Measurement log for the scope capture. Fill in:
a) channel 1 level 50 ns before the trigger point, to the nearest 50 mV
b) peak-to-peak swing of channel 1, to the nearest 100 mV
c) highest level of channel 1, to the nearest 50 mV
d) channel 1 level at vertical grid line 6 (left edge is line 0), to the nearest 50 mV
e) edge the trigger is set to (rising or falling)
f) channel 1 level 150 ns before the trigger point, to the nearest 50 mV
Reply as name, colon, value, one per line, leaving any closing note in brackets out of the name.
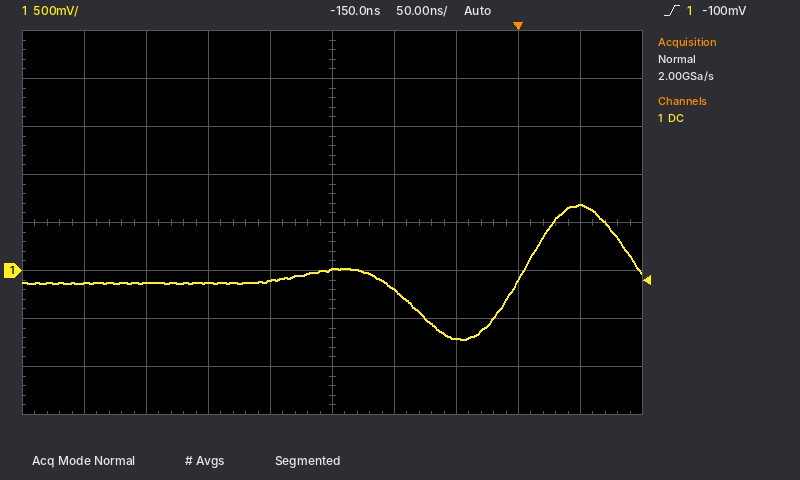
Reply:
channel 1 level 50 ns before the trigger point, to the nearest 50 mV: -700 mV
peak-to-peak swing of channel 1, to the nearest 100 mV: 1.40 V
highest level of channel 1, to the nearest 50 mV: 700 mV
channel 1 level at vertical grid line 6 (left edge is line 0), to the nearest 50 mV: -200 mV
edge the trigger is set to: rising
channel 1 level 150 ns before the trigger point, to the nearest 50 mV: 0 mV
